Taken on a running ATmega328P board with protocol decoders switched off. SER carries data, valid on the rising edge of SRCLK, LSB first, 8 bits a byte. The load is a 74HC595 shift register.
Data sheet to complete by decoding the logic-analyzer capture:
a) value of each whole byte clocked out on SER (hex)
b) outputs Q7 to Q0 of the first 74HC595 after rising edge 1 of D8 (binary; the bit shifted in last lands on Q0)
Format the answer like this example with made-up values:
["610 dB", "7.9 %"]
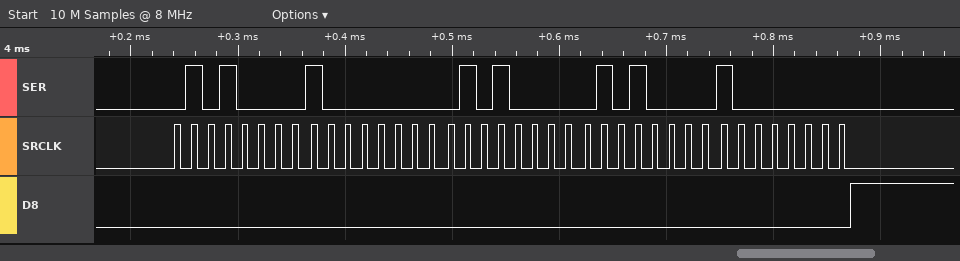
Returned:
["0A 01 0A 0A 01", "10000000"]
